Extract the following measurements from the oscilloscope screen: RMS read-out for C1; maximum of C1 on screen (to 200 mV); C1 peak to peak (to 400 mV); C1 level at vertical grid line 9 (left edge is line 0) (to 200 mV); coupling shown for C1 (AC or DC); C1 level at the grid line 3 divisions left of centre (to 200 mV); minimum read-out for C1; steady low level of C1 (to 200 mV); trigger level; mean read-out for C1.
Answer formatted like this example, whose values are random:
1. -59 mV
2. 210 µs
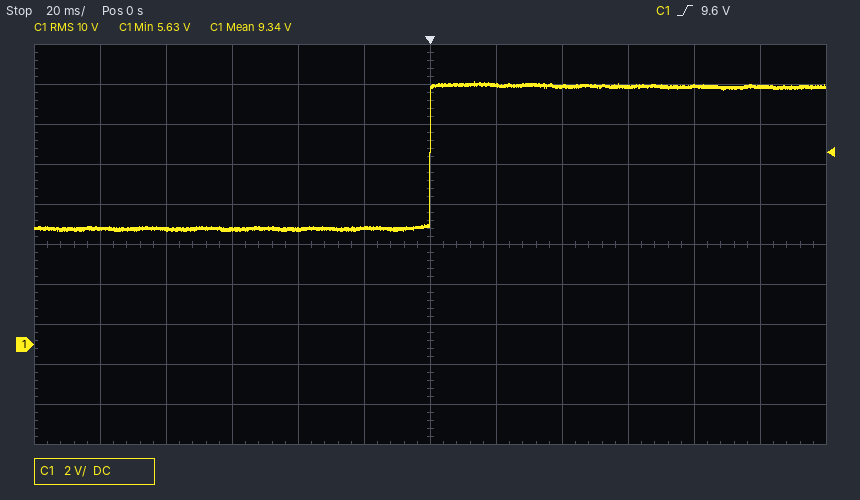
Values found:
1. 10 V
2. 13.2 V
3. 7.6 V
4. 12.8 V
5. DC
6. 5.8 V
7. 5.63 V
8. 5.8 V
9. 9.6 V
10. 9.34 V
